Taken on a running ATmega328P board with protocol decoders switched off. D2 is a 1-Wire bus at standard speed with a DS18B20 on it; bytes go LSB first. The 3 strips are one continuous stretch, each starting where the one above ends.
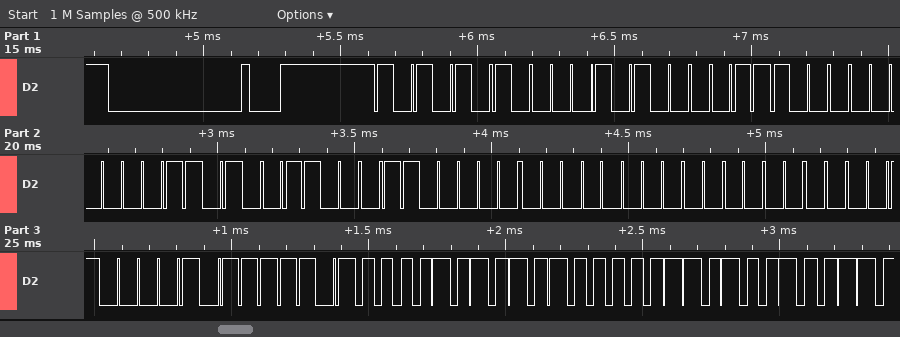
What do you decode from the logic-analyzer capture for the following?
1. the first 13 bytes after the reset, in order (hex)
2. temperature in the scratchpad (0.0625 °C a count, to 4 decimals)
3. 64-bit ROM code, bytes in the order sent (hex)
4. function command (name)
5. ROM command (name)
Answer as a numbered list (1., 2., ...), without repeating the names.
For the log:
1. 55 28 1C C0 32 06 00 00 84 BE 50 05 4B
2. 85.0000 °C
3. 28 1C C0 32 06 00 00 84
4. Read Scratchpad
5. Match ROM
